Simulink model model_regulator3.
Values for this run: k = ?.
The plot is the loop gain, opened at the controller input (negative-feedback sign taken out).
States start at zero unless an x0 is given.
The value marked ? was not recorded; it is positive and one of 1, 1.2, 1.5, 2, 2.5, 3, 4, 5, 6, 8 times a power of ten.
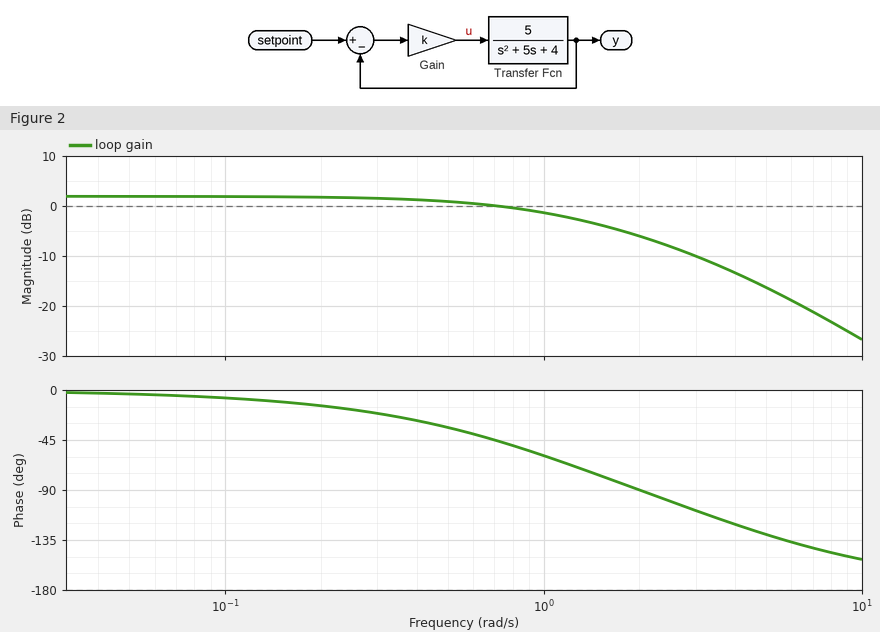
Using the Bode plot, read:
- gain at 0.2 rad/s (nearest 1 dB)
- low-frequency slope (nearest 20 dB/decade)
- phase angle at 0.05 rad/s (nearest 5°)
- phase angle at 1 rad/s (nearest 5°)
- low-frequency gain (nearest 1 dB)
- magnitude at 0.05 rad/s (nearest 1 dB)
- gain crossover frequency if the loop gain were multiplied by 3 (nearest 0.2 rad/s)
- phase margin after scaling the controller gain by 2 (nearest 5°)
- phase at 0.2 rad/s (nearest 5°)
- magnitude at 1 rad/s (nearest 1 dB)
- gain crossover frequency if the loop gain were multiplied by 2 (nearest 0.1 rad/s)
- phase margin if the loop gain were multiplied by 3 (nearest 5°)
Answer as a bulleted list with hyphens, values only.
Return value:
- 2 dB
- 0 dB/decade
- -5°
- -60°
- 2 dB
- 2 dB
- 2.8 rad/s
- 90°
- -15°
- -1 dB
- 2.0 rad/s
- 75°
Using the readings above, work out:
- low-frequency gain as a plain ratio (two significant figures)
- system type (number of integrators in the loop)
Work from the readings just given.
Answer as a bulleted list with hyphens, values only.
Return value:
- 1.3
- 0
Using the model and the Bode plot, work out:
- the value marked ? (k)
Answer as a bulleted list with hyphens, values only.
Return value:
- 1
